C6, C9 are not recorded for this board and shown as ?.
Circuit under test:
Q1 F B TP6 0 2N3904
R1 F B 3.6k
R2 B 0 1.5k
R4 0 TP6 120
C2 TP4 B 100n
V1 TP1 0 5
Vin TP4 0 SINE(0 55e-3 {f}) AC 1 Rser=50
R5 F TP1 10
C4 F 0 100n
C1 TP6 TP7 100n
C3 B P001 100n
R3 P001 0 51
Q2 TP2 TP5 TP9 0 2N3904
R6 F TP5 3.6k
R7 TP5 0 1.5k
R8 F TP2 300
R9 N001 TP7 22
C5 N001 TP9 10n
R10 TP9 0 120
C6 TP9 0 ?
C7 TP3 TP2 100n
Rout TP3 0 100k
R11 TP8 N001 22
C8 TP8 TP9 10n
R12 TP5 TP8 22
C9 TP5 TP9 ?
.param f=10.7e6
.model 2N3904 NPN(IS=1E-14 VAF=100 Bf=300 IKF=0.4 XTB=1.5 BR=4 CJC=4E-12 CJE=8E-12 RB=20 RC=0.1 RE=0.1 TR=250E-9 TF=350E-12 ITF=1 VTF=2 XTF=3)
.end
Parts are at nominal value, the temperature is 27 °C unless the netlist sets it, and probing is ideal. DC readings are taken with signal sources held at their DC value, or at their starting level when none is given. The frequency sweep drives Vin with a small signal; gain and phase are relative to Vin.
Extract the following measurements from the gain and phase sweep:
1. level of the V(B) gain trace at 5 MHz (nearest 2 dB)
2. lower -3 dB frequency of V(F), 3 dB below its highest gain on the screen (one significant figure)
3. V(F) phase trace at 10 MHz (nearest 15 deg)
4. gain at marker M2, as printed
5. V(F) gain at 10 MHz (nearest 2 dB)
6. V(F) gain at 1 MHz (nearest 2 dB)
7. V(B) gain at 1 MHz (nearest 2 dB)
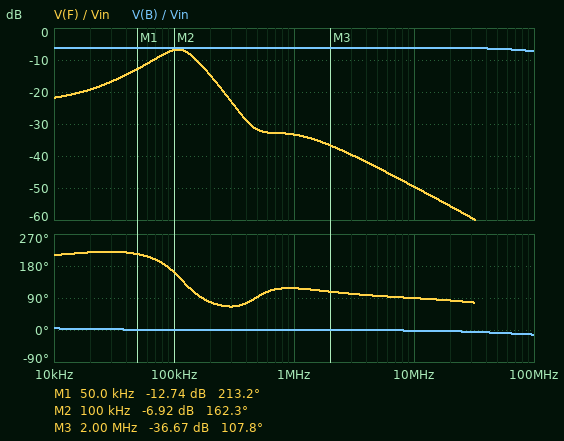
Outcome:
-6 dB
70 kHz
90 deg
-6.92 dB
-50 dB
-34 dB
-6 dB
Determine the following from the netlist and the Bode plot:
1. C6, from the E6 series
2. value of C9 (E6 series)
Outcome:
150 nF
33 nF
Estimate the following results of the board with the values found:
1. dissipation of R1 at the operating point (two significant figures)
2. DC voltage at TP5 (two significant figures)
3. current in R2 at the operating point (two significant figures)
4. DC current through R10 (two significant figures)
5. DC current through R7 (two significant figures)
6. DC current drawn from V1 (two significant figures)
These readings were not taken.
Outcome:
3.3 mW
1.4 V
940 µA
5.9 mA
940 µA
14 mA
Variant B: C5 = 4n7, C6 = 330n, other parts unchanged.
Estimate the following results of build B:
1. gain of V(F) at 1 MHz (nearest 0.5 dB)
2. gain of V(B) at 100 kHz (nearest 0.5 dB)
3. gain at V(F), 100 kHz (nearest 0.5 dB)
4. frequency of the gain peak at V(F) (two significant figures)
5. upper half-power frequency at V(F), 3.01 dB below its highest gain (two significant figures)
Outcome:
-35.5 dB
-6.0 dB
-6.0 dB
76 kHz
120 kHz
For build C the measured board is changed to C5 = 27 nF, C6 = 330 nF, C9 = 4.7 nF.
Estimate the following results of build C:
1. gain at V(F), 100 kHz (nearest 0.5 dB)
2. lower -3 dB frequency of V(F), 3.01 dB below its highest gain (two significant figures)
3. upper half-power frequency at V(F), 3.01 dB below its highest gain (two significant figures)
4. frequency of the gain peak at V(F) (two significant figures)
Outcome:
-5.5 dB
47 kHz
170 kHz
97 kHz
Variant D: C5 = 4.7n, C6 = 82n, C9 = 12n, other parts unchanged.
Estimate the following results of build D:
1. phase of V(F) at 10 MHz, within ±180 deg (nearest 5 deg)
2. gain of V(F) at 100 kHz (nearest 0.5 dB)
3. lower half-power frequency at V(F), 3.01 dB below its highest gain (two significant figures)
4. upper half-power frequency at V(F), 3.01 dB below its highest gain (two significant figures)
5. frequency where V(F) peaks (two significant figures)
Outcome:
95 deg
-13.0 dB
130 kHz
280 kHz
210 kHz
